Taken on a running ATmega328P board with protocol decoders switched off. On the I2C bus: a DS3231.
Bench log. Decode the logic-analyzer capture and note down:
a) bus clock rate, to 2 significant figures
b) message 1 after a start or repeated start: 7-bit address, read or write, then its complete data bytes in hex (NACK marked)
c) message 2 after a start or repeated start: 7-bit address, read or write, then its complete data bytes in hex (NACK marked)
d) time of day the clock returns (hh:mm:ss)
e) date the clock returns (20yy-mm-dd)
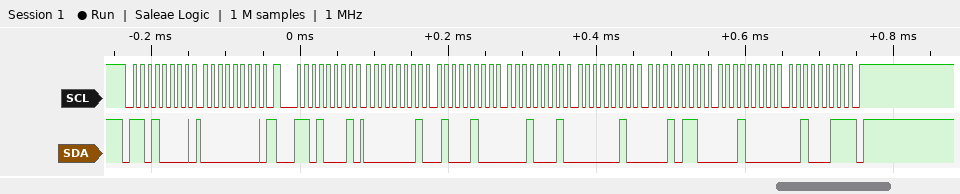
100 kHz
0x68 write: 00
0x68 read: 01 44 11 02 16 10 23 NACK
11:44:01
2023-10-16
